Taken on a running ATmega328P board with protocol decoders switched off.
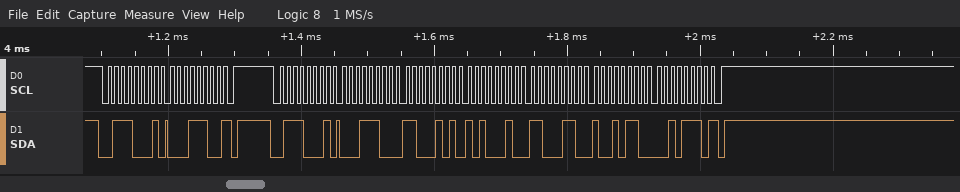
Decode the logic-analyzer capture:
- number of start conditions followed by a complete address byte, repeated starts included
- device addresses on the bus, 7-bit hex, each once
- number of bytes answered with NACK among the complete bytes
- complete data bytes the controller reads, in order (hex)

2
0x38
2
1C 1C C5 A2 C6 96 2E
